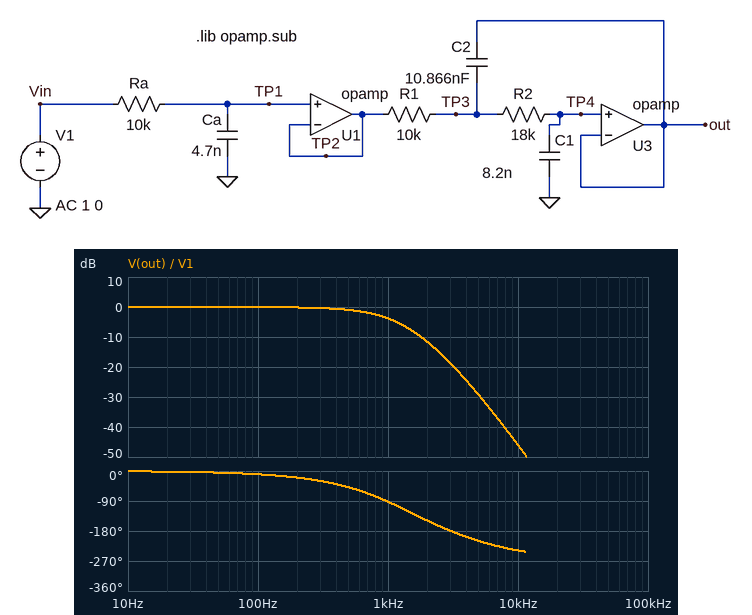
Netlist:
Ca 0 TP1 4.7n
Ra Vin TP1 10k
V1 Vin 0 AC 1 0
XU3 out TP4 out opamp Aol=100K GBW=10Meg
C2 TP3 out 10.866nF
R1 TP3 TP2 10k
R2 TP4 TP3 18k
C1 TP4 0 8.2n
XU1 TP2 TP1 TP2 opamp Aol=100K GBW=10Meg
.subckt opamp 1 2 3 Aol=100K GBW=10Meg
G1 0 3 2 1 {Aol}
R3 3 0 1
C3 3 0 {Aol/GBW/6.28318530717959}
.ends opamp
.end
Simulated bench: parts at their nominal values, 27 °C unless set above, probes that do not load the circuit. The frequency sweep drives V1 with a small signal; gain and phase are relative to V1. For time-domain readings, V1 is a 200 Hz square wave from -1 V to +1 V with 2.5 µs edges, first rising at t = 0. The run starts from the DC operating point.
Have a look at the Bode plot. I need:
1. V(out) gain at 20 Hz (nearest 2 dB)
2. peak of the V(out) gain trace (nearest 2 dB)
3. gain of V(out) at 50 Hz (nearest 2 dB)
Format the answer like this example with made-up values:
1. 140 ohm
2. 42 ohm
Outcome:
1. 0 dB
2. 0 dB
3. 0 dB
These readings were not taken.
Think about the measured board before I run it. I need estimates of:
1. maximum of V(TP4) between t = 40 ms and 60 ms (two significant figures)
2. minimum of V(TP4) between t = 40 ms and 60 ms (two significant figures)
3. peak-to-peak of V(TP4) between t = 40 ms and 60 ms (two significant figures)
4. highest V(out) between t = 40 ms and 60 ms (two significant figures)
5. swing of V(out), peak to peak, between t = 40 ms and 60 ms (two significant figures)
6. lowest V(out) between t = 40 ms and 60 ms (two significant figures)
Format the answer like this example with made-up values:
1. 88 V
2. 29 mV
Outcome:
1. 1.0 V
2. -1.0 V
3. 2.0 V
4. 1.0 V
5. 2.0 V
6. -1.0 V
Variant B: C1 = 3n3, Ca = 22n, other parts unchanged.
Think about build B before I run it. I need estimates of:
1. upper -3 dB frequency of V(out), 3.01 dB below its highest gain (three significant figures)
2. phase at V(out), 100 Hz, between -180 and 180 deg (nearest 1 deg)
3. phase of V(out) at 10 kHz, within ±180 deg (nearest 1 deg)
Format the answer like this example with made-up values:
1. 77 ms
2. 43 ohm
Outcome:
1. 785 Hz
2. -11 deg
3. 107 deg
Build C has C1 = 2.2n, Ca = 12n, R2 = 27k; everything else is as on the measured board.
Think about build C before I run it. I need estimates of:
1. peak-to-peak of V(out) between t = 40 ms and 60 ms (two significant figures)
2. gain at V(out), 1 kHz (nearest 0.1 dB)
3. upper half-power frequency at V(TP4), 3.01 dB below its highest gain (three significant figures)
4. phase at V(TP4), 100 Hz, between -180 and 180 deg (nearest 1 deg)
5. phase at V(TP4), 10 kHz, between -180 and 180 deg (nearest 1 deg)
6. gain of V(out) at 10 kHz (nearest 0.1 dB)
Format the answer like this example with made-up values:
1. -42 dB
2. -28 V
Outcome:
1. 2.1 V
2. -1.1 dB
3. 1.63 kHz
4. -7 deg
5. 109 deg
6. -45.6 dB
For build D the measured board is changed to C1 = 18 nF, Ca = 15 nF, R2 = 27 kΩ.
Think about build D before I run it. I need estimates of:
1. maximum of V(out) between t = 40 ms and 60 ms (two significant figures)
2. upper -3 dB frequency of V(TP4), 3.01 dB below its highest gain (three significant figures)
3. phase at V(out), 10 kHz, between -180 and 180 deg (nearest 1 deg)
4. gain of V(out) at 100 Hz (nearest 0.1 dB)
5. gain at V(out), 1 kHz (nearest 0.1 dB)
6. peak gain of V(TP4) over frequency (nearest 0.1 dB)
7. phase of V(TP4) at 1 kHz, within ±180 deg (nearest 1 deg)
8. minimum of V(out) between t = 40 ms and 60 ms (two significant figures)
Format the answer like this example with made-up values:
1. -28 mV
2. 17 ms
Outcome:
1. 960 mV
2. 256 Hz
3. 107 deg
4. -0.6 dB
5. -15.5 dB
6. 0 dB
7. -148 deg
8. -960 mV
